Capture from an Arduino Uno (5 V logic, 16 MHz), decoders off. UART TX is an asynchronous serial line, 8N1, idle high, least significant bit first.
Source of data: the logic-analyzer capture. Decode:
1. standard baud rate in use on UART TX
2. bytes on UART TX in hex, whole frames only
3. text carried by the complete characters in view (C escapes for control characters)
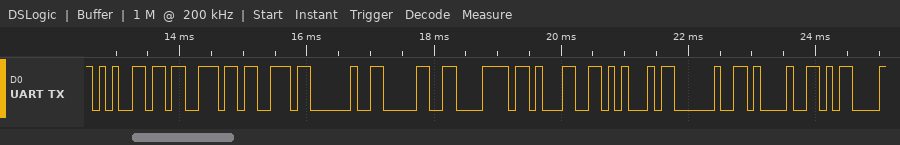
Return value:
9600 baud
65 73 73 20 30 78 31 45 20 21 0D
"ess 0x1E !\r"
